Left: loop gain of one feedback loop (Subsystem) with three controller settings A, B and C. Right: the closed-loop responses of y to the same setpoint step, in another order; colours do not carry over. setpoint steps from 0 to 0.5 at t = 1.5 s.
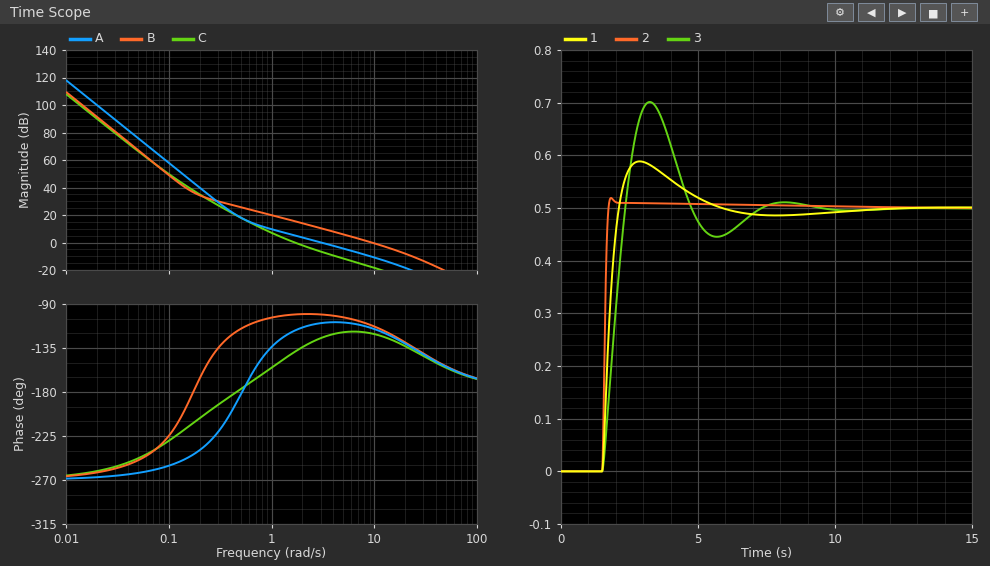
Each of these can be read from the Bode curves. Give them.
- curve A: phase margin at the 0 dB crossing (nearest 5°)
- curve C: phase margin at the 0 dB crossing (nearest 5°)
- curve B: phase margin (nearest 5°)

70°
40°
70°
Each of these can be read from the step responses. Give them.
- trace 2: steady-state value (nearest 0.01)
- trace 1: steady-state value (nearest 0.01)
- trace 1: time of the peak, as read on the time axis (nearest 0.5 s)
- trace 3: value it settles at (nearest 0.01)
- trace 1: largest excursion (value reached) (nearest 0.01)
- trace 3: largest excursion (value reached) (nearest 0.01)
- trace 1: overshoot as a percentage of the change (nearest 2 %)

0.50
0.50
3.0 s
0.50
0.59
0.70
18 %
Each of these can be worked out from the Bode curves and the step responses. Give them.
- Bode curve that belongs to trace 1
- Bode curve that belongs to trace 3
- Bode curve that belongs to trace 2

A
C
B
